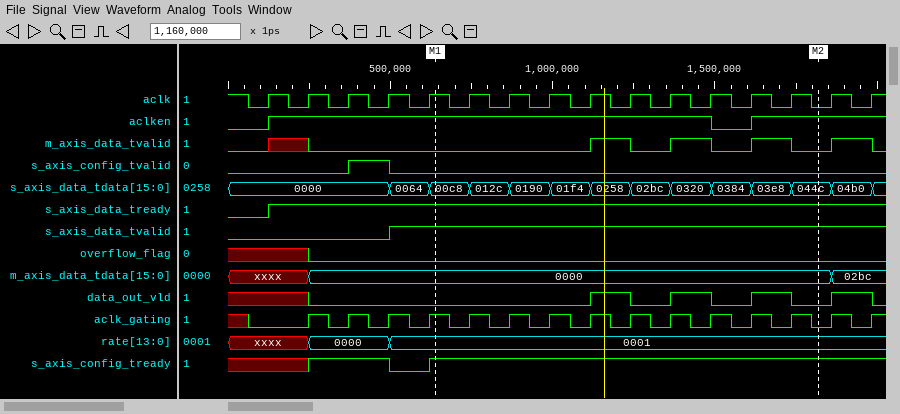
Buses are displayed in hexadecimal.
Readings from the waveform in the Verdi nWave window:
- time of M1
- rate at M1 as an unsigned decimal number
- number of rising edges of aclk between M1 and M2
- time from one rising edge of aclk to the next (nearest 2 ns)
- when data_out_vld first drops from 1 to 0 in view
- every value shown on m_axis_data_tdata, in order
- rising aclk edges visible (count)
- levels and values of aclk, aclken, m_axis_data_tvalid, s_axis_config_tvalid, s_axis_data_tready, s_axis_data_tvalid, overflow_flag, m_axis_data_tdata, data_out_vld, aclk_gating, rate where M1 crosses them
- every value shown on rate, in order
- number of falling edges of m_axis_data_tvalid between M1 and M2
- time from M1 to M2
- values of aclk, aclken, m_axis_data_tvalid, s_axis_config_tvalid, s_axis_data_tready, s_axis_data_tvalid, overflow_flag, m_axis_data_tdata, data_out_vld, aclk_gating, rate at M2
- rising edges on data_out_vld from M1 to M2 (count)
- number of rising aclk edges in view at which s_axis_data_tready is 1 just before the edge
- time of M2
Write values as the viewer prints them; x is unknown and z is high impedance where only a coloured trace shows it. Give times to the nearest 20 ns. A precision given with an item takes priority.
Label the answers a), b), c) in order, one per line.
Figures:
a) 640 ns
b) 1
c) 9
d) 124 ns
e) 1240 ns
f) xxxx, 0000, 02bc
g) 16
h) aclk=1, aclken=1, m_axis_data_tvalid=0, s_axis_config_tvalid=0, s_axis_data_tready=1, s_axis_data_tvalid=1, overflow_flag=0, m_axis_data_tdata=0000, data_out_vld=0, aclk_gating=1, rate=0001
i) xxxx, 0000, 0001
j) 3
k) 1180 ns
l) aclk=0, aclken=1, m_axis_data_tvalid=0, s_axis_config_tvalid=0, s_axis_data_tready=1, s_axis_data_tvalid=1, overflow_flag=0, m_axis_data_tdata=0000, data_out_vld=0, aclk_gating=0, rate=0001
m) 3
n) 15
o) 1820 ns
